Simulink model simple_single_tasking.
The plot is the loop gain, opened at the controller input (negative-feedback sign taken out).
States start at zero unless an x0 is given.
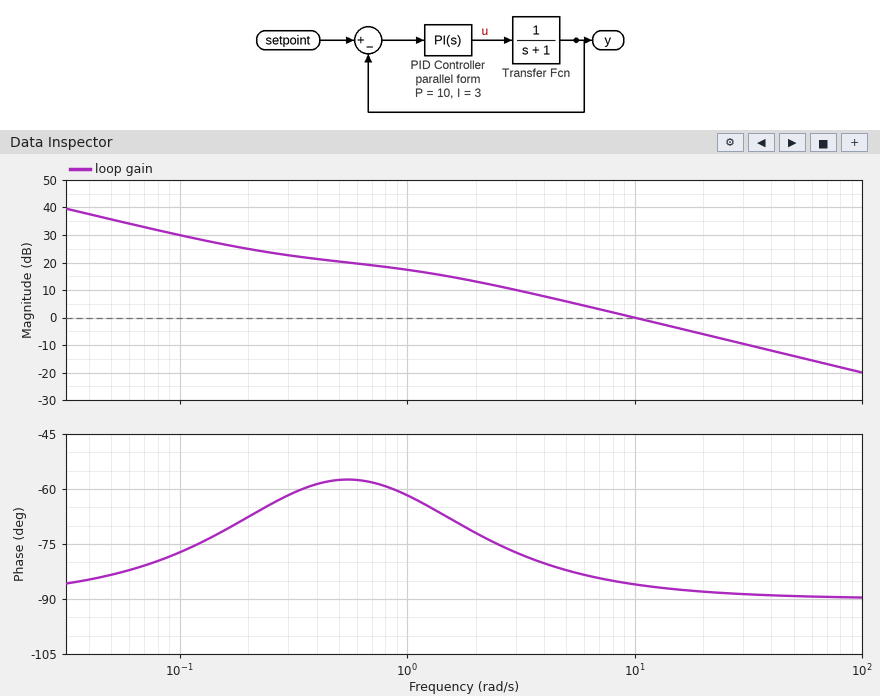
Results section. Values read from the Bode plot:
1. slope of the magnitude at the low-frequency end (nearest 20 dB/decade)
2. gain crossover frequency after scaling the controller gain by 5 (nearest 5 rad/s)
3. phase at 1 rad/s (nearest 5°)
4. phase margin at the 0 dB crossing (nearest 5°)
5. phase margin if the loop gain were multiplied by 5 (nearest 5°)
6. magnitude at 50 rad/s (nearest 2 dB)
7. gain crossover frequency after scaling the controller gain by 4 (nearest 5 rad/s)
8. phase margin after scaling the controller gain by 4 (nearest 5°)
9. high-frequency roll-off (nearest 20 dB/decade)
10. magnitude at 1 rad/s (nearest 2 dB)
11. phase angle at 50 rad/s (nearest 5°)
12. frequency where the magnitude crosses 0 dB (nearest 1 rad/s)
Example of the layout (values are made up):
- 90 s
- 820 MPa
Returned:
- -20 dB/decade
- 50 rad/s
- -60°
- 95°
- 90°
- -14 dB
- 40 rad/s
- 90°
- -20 dB/decade
- 18 dB
- -90°
- 10 rad/s
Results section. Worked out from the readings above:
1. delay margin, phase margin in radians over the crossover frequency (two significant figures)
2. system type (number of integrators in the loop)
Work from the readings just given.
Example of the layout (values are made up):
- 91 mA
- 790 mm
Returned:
- 0.17 s
- 1
